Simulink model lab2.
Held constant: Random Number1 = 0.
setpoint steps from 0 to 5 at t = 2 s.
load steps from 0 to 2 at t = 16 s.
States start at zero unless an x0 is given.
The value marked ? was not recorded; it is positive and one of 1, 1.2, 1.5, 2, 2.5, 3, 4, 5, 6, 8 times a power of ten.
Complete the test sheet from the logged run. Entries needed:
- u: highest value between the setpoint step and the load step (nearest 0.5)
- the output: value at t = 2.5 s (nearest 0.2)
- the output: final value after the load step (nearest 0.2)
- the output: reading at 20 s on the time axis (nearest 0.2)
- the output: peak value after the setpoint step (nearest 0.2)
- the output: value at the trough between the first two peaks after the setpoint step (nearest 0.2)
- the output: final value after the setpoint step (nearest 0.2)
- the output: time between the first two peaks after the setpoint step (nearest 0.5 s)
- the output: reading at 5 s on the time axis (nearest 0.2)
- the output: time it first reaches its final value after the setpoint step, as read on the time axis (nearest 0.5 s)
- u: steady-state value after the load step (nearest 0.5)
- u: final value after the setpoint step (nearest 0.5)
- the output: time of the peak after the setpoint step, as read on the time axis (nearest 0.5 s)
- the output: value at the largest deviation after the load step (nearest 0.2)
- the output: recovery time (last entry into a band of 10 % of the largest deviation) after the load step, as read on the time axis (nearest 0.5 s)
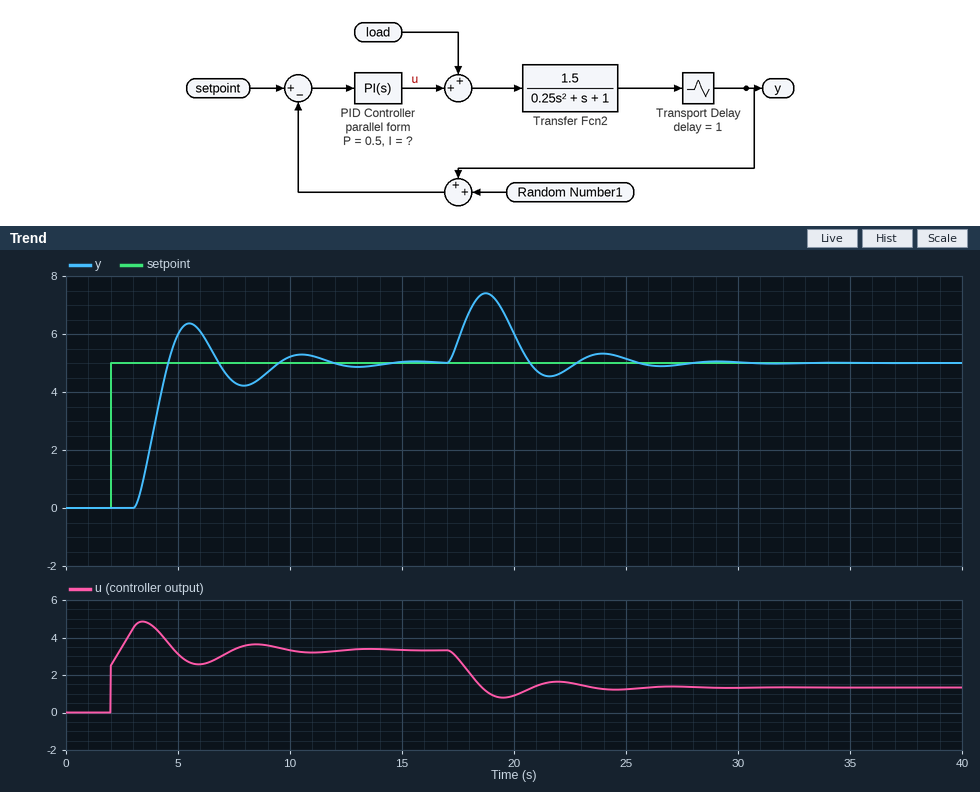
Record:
5.0
0.0
5.0
6.0
6.4
4.2
5.0
5.0 s
6.0
4.5 s
1.5
3.5
5.5 s
7.4
24.5 s
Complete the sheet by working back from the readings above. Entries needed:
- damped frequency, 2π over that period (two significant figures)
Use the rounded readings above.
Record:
1.3 rad/s
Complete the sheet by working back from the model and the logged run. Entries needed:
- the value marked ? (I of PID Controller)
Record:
0.4
